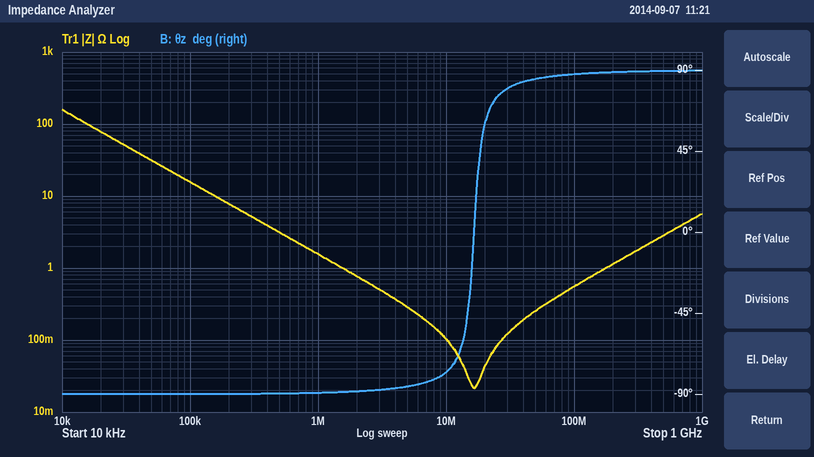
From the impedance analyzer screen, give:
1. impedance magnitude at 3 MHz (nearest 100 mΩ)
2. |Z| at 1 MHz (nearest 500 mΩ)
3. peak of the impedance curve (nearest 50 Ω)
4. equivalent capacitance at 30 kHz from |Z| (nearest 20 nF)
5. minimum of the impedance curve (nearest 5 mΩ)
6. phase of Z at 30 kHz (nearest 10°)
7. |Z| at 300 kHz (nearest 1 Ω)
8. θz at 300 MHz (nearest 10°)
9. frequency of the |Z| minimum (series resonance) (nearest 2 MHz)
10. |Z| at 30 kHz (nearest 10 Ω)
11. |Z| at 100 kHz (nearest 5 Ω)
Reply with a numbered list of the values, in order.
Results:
1. 500 mΩ
2. 1.5 Ω
3. 150 Ω
4. 100 nF
5. 20 mΩ
6. -90°
7. 5 Ω
8. 90°
9. 16 MHz
10. 50 Ω
11. 15 Ω
